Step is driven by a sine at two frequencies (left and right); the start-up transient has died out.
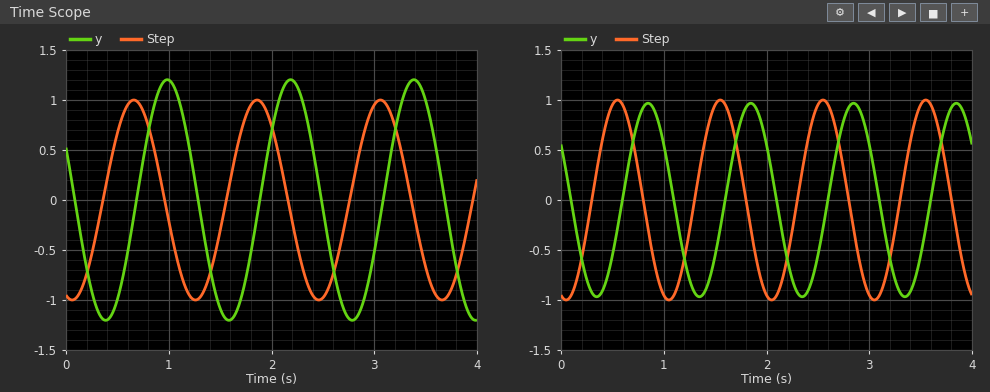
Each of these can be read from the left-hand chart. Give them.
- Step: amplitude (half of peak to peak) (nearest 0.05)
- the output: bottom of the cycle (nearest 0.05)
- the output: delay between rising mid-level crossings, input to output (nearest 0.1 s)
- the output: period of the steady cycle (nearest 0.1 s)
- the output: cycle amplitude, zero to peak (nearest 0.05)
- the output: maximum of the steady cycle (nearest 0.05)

1.00
-1.20
0.3 s
1.2 s
1.20
1.20
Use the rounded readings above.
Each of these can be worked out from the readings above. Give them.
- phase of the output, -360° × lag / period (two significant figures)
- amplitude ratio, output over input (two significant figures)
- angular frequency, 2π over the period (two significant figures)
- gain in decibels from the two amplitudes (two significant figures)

-90°
1.2
5.2 rad/s
1.6 dB
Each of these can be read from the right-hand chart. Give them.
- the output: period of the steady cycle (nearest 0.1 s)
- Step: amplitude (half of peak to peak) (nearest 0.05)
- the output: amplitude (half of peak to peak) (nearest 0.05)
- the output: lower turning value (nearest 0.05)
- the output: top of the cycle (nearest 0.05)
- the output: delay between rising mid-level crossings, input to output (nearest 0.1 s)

1.0 s
1.00
0.95
-0.95
0.95
0.3 s
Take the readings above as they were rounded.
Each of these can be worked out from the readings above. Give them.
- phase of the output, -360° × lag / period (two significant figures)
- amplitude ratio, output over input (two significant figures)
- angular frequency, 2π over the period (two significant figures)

-110°
0.95
6.3 rad/s
